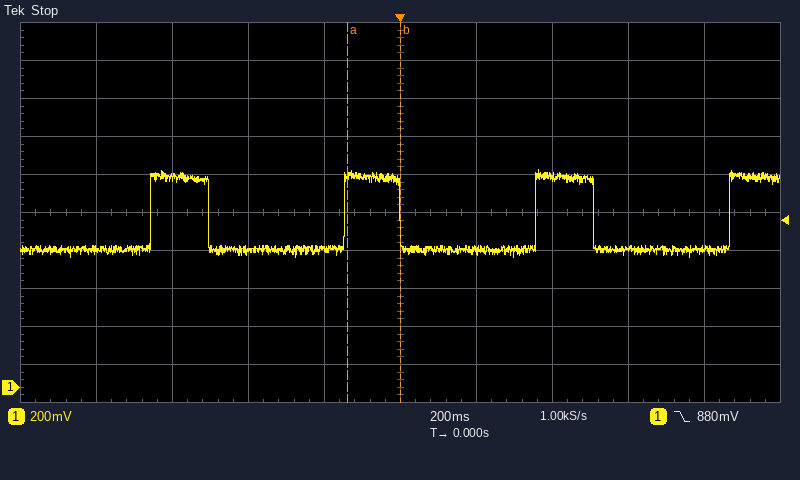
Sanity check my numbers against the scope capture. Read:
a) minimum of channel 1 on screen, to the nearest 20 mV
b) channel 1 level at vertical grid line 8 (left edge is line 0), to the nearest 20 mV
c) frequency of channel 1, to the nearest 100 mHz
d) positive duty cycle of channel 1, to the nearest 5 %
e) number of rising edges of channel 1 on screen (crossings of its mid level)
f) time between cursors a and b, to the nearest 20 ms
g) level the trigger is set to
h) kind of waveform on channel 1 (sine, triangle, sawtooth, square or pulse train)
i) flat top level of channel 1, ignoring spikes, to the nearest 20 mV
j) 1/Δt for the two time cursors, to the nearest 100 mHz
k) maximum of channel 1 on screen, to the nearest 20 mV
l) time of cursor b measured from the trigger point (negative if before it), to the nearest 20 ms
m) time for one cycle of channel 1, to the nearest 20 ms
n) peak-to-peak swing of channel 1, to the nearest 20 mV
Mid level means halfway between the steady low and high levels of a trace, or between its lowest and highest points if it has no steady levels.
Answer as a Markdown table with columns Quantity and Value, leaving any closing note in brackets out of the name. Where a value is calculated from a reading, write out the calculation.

| Quantity | Value |
|---|---|
| minimum of channel 1 on screen, to the nearest 20 mV | 680 mV |
| channel 1 level at vertical grid line 8 (left edge is line 0), to the nearest 20 mV | 740 mV |
| frequency of channel 1, to the nearest 100 mHz | 1 / 500 ms ≈ 2.0 Hz |
| positive duty cycle of channel 1, to the nearest 5 % | 30 % |
| number of rising edges of channel 1 on screen | 4 |
| time between cursors a and b, to the nearest 20 ms | 140 ms |
| level the trigger is set to | 880 mV |
| kind of waveform on channel 1 | pulse train |
| flat top level of channel 1, ignoring spikes, to the nearest 20 mV | 1.10 V |
| 1/Δt for the two time cursors, to the nearest 100 mHz | 1 / 140 ms ≈ 7.1 Hz |
| maximum of channel 1 on screen, to the nearest 20 mV | 1.14 V |
| time of cursor b measured from the trigger point (negative if before it), to the nearest 20 ms | 0 ms |
| time for one cycle of channel 1, to the nearest 20 ms | 500 ms |
| peak-to-peak swing of channel 1, to the nearest 20 mV | 1.14 V − (680 mV) = 460 mV |
